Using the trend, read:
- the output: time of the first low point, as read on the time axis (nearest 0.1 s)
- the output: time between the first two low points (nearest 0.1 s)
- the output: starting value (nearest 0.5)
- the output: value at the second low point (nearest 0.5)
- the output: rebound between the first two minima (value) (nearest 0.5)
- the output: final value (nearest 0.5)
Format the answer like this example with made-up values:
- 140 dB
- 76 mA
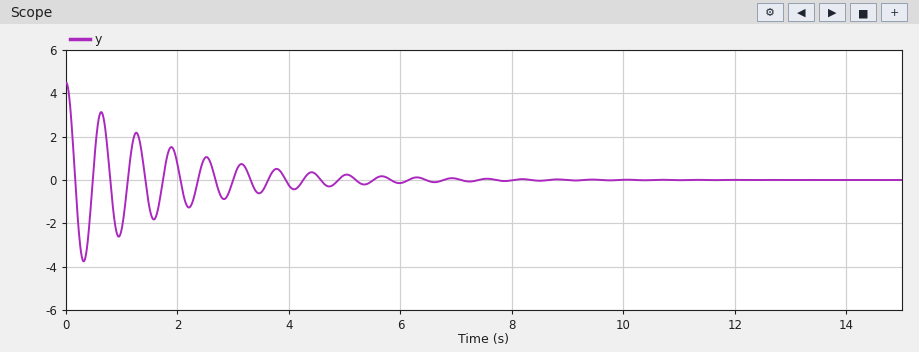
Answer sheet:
- 0.3 s
- 0.6 s
- 4.5
- -2.5
- 3.0
- 0.0
